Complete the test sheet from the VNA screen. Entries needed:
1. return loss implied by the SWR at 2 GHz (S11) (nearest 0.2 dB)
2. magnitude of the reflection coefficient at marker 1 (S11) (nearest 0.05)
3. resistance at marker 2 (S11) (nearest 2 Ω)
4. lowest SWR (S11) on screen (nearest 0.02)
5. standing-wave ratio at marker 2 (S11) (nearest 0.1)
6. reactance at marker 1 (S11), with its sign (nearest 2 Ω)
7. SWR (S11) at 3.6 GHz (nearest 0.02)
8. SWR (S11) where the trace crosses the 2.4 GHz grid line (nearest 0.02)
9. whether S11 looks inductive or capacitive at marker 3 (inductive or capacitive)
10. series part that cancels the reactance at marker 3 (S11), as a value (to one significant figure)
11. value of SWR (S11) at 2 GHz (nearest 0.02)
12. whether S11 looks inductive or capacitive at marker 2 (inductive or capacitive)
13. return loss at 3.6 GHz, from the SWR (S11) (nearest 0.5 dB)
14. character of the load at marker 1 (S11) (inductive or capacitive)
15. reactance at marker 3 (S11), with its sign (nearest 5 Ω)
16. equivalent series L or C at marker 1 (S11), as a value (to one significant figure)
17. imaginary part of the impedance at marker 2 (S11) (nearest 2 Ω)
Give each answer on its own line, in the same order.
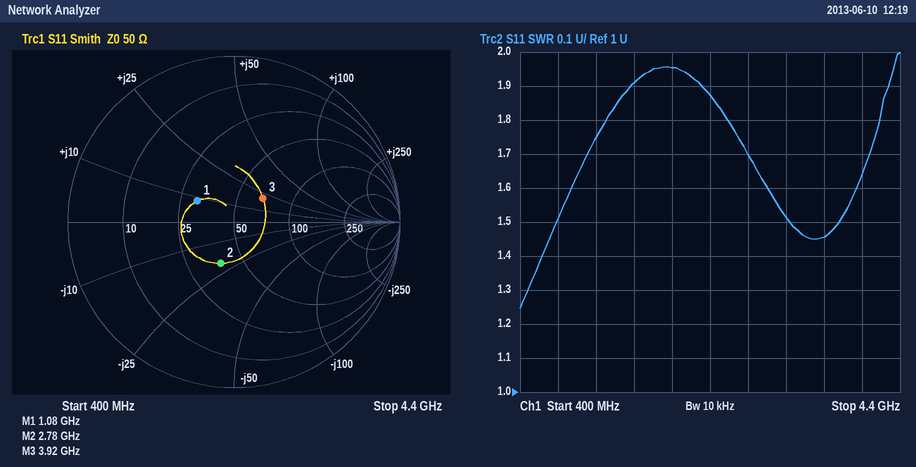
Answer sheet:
9.8 dB
0.25
38 Ω
1.24
1.7
+8 Ω
1.46
1.88
inductive
2 pF
1.96
capacitive
14.5 dB
inductive
+20 Ω
1 nH
-20 Ω
